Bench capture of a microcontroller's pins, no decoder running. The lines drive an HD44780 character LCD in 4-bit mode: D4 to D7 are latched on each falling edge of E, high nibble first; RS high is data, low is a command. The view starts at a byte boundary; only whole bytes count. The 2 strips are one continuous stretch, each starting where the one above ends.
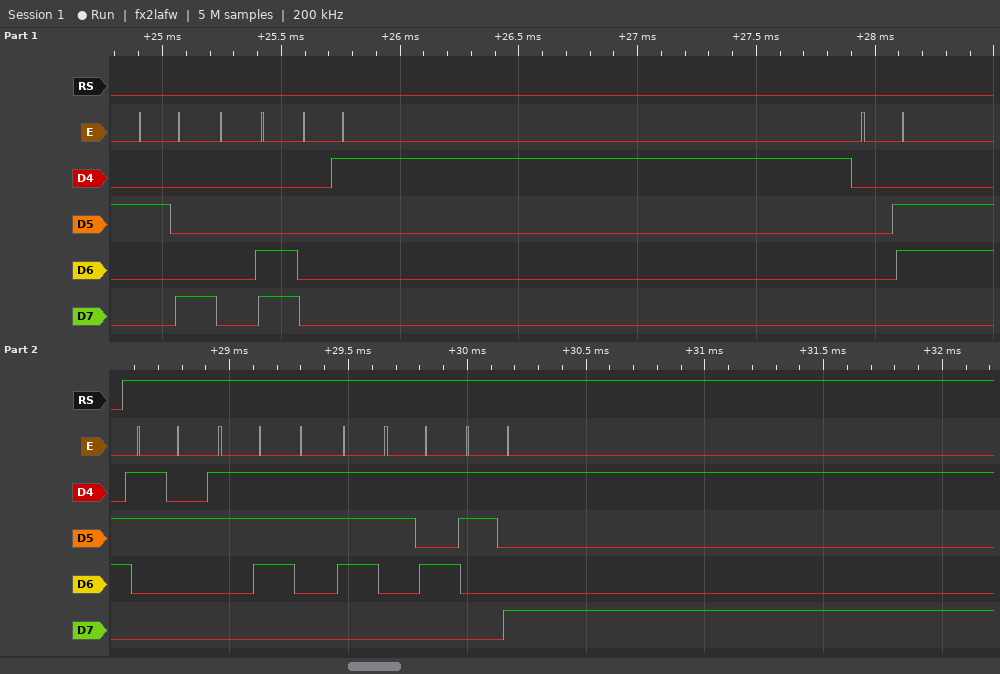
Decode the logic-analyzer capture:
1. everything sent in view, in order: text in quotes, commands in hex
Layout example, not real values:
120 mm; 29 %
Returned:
0x28 0x0C 0x01 0x06 "27759"
